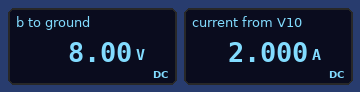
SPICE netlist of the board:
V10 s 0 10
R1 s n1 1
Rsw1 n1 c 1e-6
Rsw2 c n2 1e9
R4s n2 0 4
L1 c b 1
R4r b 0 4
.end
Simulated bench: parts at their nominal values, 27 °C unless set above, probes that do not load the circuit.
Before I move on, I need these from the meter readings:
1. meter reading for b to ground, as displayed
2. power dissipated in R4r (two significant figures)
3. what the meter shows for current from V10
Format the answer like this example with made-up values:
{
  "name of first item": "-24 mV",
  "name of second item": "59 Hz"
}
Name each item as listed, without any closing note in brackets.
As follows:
{
  "meter reading for b to ground, as displayed": "8.00 V",
  "power dissipated in R4r": "16 W",
  "what the meter shows for current from V10": "2.000 A"
}
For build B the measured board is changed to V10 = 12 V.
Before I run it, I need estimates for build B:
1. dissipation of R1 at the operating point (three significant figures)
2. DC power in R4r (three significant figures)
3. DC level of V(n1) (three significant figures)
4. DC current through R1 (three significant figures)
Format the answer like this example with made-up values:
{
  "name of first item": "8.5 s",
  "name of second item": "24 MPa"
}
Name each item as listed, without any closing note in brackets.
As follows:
{
  "dissipation of R1 at the operating point": "5.76 W",
  "DC power in R4r": "23.0 W",
  "DC level of V(n1)": "9.60 V",
  "DC current through R1": "2.40 A"
}
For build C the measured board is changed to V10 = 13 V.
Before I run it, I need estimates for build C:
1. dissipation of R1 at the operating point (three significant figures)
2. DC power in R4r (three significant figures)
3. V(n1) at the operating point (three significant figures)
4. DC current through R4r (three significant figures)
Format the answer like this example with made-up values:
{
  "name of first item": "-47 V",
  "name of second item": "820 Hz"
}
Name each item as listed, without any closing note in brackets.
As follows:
{
  "dissipation of R1 at the operating point": "6.76 W",
  "DC power in R4r": "27.0 W",
  "V(n1) at the operating point": "10.4 V",
  "DC current through R4r": "2.60 A"
}
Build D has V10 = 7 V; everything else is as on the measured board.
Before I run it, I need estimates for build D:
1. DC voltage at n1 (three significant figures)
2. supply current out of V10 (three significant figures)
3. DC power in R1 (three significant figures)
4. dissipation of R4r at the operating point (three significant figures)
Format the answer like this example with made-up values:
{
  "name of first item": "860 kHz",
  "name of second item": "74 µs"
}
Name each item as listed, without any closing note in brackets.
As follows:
{
  "DC voltage at n1": "5.60 V",
  "supply current out of V10": "1.40 A",
  "DC power in R1": "1.96 W",
  "dissipation of R4r at the operating point": "7.84 W"
}
